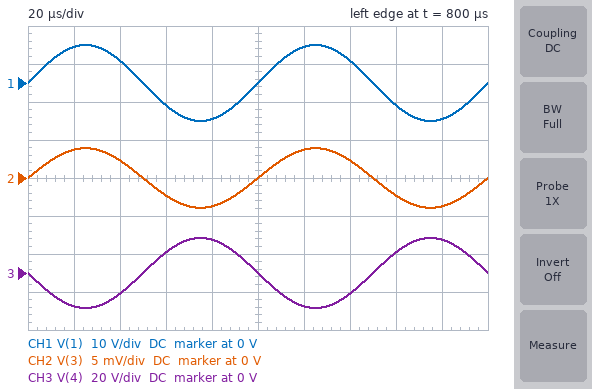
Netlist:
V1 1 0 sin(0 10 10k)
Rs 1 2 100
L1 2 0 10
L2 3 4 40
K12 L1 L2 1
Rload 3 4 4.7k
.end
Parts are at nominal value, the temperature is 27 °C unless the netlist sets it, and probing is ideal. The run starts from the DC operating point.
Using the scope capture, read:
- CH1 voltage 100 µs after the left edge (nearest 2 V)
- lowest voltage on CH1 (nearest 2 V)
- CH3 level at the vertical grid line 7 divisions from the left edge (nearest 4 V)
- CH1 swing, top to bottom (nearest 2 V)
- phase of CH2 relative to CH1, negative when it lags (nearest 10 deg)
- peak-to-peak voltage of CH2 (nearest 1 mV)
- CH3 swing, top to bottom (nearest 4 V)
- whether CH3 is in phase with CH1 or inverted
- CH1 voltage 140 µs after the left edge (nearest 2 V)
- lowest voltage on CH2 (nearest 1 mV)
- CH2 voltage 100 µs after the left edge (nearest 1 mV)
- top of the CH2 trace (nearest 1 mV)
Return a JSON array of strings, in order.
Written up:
["0 V", "-10 V", "-12 V", "20 V", "0 deg", "8 mV", "36 V", "inverted", "6 V", "-4 mV", "0 V", "4 mV"]
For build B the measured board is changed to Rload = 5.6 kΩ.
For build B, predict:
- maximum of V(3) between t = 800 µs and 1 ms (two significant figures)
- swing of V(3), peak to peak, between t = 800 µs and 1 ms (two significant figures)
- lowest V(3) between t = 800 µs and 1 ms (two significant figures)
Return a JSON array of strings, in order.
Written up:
["3.3 mV", "6.7 mV", "-3.3 mV"]
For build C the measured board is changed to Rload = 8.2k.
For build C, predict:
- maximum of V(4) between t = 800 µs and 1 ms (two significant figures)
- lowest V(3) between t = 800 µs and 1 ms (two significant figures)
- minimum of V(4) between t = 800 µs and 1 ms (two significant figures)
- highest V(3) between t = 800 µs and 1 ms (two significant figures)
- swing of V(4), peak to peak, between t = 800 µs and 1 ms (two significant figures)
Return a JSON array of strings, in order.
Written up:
["19 V", "-2.3 mV", "-19 V", "2.3 mV", "38 V"]
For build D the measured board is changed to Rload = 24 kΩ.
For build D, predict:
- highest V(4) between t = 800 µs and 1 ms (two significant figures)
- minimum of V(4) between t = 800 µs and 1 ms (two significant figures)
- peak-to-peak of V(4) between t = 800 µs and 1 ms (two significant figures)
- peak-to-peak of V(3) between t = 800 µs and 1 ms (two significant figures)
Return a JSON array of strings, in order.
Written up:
["20 V", "-20 V", "39 V", "1.6 mV"]
